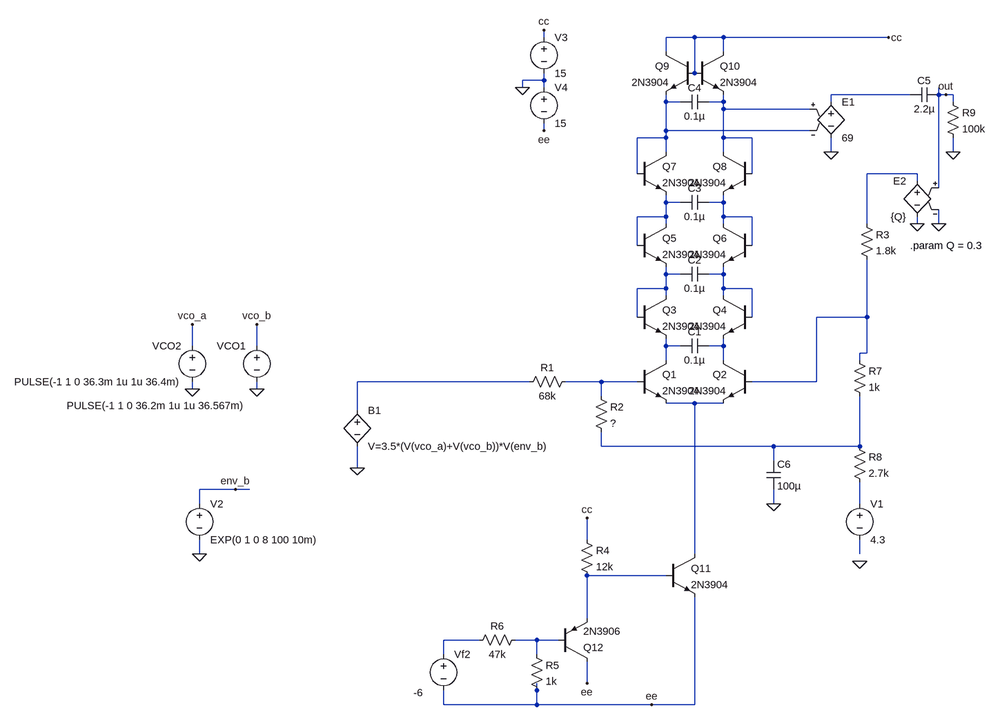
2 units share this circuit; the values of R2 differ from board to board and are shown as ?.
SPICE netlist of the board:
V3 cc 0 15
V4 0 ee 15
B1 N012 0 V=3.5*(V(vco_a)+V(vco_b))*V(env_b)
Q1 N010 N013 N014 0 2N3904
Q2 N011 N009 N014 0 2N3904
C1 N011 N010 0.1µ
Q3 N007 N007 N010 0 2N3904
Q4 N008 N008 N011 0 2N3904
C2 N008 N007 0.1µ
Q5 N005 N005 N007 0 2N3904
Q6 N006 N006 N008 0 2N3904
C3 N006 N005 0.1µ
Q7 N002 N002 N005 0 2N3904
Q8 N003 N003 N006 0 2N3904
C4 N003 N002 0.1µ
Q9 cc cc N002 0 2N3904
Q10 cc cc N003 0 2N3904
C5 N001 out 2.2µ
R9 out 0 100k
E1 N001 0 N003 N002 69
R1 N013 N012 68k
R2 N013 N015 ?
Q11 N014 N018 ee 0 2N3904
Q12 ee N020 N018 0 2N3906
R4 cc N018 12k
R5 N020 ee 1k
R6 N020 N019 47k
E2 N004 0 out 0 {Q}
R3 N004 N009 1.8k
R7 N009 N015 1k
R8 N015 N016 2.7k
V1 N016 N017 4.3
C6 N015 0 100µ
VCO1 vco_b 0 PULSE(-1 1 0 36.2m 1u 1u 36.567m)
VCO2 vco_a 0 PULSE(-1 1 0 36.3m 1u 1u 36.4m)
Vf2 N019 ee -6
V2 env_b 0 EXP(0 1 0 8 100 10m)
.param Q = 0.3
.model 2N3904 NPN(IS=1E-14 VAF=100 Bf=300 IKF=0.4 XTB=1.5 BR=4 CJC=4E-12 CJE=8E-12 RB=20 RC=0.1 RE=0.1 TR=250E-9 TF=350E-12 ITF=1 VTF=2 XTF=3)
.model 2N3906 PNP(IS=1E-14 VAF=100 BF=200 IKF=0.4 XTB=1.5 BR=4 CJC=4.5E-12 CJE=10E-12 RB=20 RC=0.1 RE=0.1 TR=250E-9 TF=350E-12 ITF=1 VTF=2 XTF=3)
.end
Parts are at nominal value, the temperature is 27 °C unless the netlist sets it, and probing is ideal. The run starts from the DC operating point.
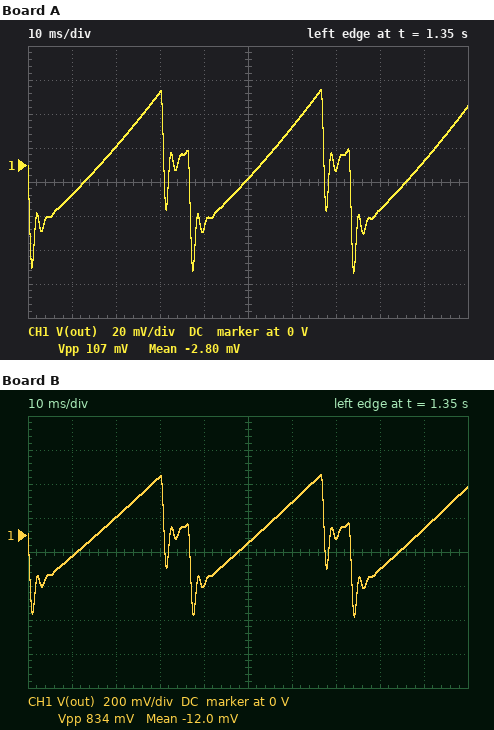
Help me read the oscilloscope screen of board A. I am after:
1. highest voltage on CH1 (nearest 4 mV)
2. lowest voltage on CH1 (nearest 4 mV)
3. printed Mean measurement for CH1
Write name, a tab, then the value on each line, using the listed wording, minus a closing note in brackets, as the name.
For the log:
highest voltage on CH1	44 mV
lowest voltage on CH1	-64 mV
printed Mean measurement for CH1	-2.80 mV
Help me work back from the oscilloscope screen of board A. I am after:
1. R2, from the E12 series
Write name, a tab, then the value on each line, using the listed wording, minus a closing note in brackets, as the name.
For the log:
R2, from the E12 series	390 Ω
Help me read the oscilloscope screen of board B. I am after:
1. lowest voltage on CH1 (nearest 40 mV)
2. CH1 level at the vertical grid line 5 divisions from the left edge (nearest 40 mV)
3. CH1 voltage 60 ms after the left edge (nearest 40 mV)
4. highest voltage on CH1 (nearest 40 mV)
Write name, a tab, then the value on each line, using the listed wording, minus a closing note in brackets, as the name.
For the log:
lowest voltage on CH1	-480 mV
CH1 level at the vertical grid line 5 divisions from the left edge	-40 mV
CH1 voltage 60 ms after the left edge	200 mV
highest voltage on CH1	360 mV
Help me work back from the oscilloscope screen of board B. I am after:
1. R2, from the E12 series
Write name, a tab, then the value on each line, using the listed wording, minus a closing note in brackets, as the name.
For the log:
R2, from the E12 series	3.3 kΩ
